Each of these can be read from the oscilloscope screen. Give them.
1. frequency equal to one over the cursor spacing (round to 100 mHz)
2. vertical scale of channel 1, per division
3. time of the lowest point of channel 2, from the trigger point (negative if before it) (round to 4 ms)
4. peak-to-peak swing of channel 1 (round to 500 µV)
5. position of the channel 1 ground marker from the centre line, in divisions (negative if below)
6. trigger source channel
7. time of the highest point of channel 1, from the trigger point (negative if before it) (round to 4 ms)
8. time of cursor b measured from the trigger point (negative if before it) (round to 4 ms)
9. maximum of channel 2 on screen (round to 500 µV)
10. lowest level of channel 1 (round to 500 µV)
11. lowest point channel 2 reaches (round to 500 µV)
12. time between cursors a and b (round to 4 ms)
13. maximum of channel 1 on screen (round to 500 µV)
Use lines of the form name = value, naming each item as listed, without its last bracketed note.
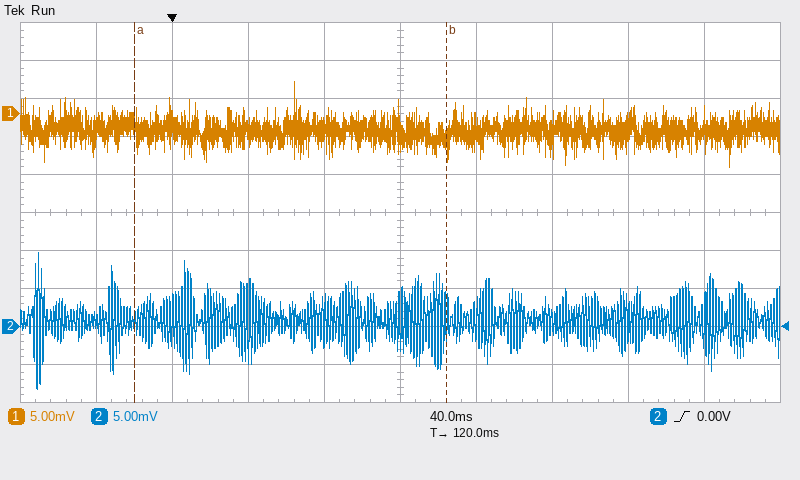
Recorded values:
frequency equal to one over the cursor spacing = 6.1 Hz
vertical scale of channel 1, per division = 5 mV
time of the lowest point of channel 2, from the trigger point (negative if before it) = -72 ms
peak-to-peak swing of channel 1 = 11.0 mV
position of the channel 1 ground marker from the centre line, in divisions = +2.6 div
trigger source channel = channel 2
time of the highest point of channel 1, from the trigger point (negative if before it) = +64 ms
time of cursor b measured from the trigger point (negative if before it) = +144 ms
maximum of channel 2 on screen = 9.5 mV
lowest level of channel 1 = -7.0 mV
lowest point channel 2 reaches = -8.0 mV
time between cursors a and b = 164 ms
maximum of channel 1 on screen = 4.0 mV
